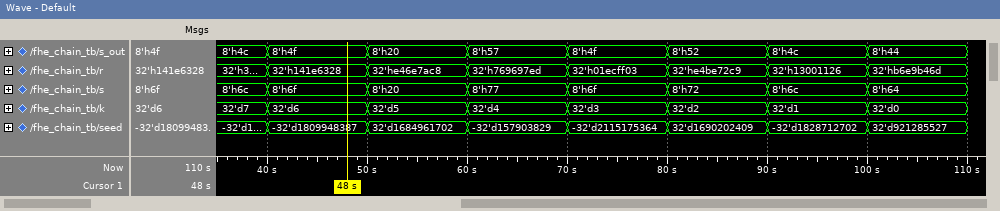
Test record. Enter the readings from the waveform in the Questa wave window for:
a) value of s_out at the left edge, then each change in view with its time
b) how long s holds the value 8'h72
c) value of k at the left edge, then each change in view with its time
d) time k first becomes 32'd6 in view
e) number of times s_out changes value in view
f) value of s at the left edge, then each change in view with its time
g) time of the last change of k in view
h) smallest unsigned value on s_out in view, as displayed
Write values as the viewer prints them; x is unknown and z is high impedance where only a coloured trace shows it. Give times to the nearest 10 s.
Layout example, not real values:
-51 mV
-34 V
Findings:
8'h4c, 8'h4f at 40 s, 8'h20 at 50 s, 8'h57 at 60 s, 8'h4f at 70 s, 8'h52 at 80 s, 8'h4c at 90 s, 8'h44 at 100 s
10 s
32'd7, 32'd6 at 40 s, 32'd5 at 50 s, 32'd4 at 60 s, 32'd3 at 70 s, 32'd2 at 80 s, 32'd1 at 90 s, 32'd0 at 100 s
40 s
7
8'h6c, 8'h6f at 40 s, 8'h20 at 50 s, 8'h77 at 60 s, 8'h6f at 70 s, 8'h72 at 80 s, 8'h6c at 90 s, 8'h64 at 100 s
100 s
8'h20
